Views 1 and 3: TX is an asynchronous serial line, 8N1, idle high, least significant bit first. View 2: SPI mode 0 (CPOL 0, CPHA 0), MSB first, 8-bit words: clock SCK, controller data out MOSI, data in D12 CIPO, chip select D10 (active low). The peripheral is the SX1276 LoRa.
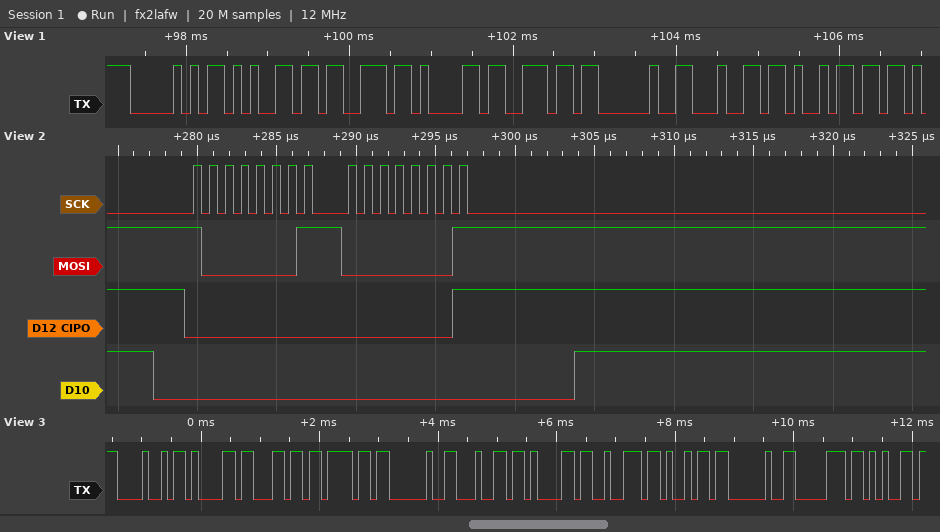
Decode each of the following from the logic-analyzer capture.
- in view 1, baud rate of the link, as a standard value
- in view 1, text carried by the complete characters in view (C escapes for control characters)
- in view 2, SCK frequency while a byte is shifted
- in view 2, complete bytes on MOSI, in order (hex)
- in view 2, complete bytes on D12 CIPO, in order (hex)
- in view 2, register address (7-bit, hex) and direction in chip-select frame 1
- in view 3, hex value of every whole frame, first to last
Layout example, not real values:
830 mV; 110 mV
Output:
9600 baud; "Pesan di"; 1 MHz; 81 01; 00 01; 0x01 write; 48 61 6C 6F 20 64 61 72 69 20 70 65
